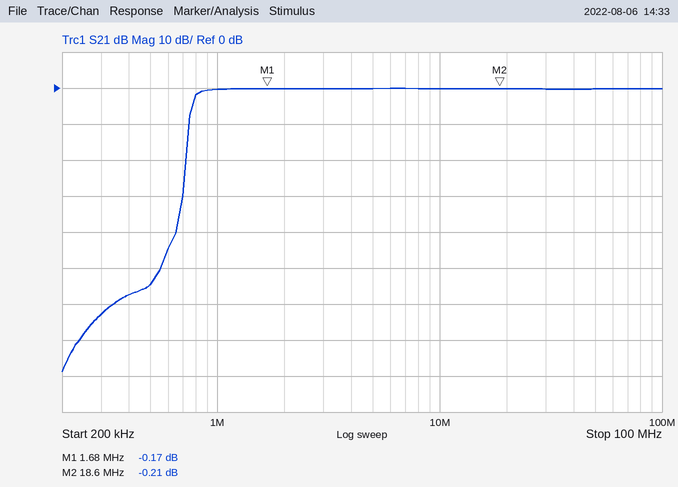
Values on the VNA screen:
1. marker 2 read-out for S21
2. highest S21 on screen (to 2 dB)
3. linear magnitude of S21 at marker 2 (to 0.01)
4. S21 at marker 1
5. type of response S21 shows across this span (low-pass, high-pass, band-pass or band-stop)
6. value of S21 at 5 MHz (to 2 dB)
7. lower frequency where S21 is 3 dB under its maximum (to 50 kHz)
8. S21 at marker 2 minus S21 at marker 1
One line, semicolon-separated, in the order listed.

-0.21 dB; 0 dB; 0.98; -0.17 dB; high-pass; 0 dB; 800 kHz; -0.04 dB
